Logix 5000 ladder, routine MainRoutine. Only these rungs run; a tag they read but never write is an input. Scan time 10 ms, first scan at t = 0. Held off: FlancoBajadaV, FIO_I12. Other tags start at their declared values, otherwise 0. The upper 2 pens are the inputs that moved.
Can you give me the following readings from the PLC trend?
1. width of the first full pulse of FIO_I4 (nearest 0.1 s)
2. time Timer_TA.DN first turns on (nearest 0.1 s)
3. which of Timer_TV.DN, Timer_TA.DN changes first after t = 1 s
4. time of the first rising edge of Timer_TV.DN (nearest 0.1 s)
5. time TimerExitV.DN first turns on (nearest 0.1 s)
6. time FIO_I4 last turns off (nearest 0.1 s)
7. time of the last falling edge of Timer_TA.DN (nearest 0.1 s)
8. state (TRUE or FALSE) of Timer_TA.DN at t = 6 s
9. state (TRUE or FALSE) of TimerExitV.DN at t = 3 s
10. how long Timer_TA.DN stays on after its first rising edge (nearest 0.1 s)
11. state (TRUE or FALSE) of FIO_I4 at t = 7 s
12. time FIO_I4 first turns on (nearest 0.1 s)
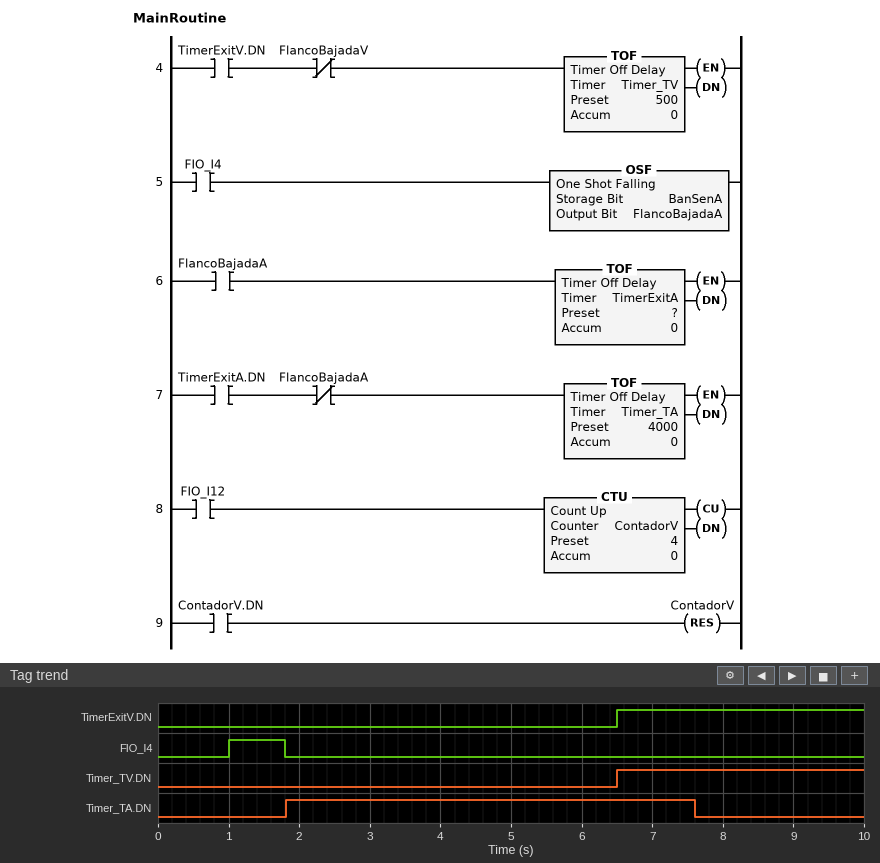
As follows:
0.8 s
1.8 s
Timer_TA.DN
6.5 s
6.5 s
1.8 s
7.6 s
TRUE
FALSE
5.8 s
FALSE
1.0 s
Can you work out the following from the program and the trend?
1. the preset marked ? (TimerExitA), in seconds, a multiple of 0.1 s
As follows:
1.8 s
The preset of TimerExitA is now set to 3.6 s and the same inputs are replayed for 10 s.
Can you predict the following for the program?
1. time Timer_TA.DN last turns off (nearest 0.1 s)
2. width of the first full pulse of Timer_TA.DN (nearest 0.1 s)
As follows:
9.4 s
7.6 s
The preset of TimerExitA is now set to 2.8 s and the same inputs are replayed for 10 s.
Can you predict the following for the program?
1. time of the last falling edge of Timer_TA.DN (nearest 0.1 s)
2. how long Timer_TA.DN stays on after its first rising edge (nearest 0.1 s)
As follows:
8.6 s
6.8 s
